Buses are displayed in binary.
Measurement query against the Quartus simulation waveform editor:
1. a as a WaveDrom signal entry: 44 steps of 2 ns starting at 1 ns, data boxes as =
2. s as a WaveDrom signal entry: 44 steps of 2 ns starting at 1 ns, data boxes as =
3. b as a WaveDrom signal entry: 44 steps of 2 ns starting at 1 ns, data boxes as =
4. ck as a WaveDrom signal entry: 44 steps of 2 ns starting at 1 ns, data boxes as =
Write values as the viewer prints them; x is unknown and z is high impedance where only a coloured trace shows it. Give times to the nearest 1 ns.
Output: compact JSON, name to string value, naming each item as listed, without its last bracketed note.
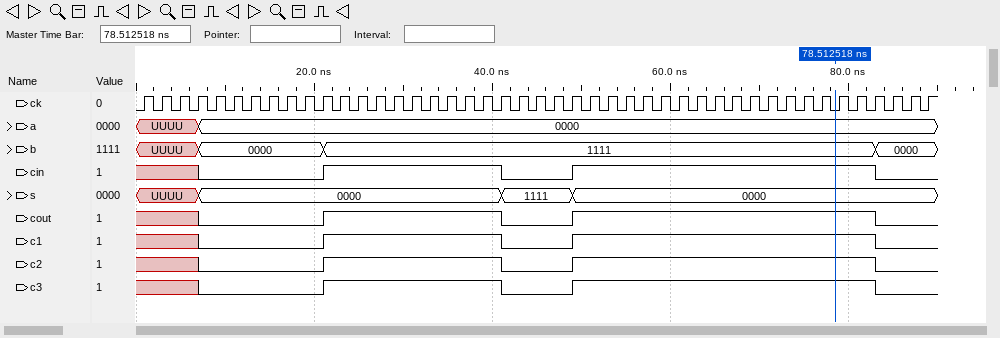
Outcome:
{"a as a WaveDrom signal entry: 44 steps of 2 ns starting at 1 ns, data boxes as =": "{name: 'a', wave: 'x..=........................................', data: '0000'}", "s as a WaveDrom signal entry: 44 steps of 2 ns starting at 1 ns, data boxes as =": "{name: 's', wave: 'x..=................=...=...................', data: '0000 1111 0000'}", "b as a WaveDrom signal entry: 44 steps of 2 ns starting at 1 ns, data boxes as =": "{name: 'b', wave: 'x..=......=..............................=..', data: '0000 1111 0000'}", "ck as a WaveDrom signal entry: 44 steps of 2 ns starting at 1 ns, data boxes as =": "{name: 'ck', wave: 'p...........................................'}"}
